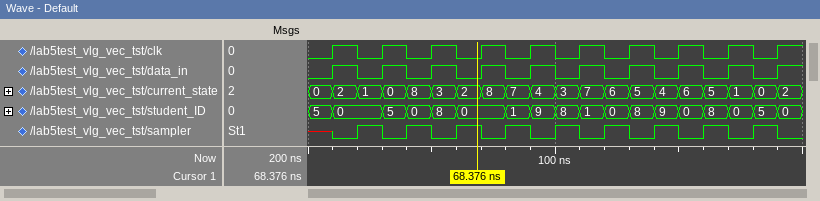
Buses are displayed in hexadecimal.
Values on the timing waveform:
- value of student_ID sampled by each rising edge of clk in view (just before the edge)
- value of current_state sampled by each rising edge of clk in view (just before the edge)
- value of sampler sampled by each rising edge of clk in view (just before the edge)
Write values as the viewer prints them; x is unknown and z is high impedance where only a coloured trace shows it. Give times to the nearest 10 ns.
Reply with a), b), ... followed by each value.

a) 5, 0, 0, 0, 1, 8, 0, 9, 8, 5
b) 0, 1, 8, 2, 7, 3, 6, 4, 5, 0
c) x 1 1 1 1 1 1 1 1 1
